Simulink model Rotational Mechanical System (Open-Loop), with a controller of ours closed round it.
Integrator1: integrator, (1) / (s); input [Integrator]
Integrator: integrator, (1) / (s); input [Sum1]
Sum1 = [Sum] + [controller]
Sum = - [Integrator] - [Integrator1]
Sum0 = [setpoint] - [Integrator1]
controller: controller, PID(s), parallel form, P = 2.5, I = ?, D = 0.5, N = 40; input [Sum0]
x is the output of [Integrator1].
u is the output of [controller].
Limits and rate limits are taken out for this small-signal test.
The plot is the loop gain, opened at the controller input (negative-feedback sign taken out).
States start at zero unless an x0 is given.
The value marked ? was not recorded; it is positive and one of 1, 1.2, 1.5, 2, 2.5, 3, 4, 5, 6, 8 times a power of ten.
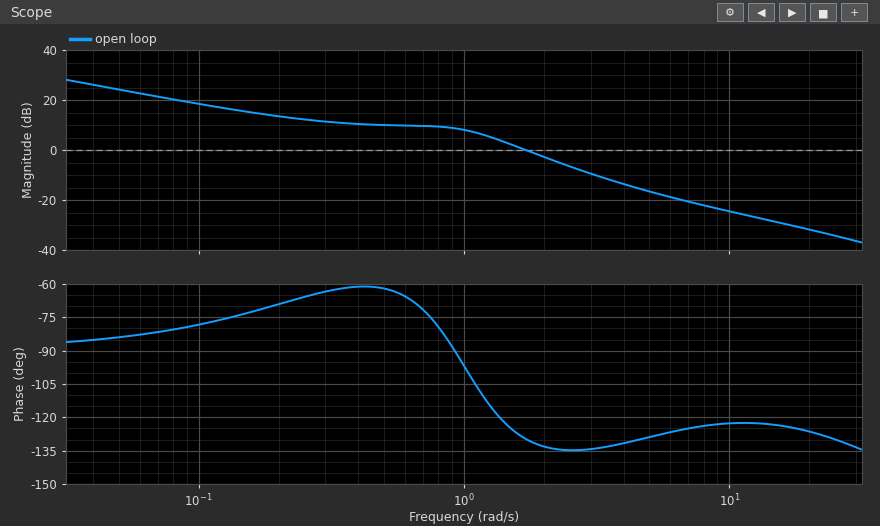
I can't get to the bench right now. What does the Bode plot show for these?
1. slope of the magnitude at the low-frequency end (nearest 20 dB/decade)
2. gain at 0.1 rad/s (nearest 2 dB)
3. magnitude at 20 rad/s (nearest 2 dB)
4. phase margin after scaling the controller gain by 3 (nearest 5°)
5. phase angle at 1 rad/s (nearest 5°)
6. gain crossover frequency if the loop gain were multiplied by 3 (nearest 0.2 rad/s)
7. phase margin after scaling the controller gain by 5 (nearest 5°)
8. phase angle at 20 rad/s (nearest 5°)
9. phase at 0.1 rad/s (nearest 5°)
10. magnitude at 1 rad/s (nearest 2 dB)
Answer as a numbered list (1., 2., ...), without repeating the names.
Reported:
1. -20 dB/decade
2. 18 dB
3. -32 dB
4. 45°
5. -95°
6. 3.0 rad/s
7. 50°
8. -125°
9. -80°
10. 8 dB
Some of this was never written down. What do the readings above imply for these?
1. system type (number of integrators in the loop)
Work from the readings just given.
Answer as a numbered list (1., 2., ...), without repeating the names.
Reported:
1. 1
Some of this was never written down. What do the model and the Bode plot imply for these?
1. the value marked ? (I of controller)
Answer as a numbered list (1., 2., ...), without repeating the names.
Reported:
1. 0.8
